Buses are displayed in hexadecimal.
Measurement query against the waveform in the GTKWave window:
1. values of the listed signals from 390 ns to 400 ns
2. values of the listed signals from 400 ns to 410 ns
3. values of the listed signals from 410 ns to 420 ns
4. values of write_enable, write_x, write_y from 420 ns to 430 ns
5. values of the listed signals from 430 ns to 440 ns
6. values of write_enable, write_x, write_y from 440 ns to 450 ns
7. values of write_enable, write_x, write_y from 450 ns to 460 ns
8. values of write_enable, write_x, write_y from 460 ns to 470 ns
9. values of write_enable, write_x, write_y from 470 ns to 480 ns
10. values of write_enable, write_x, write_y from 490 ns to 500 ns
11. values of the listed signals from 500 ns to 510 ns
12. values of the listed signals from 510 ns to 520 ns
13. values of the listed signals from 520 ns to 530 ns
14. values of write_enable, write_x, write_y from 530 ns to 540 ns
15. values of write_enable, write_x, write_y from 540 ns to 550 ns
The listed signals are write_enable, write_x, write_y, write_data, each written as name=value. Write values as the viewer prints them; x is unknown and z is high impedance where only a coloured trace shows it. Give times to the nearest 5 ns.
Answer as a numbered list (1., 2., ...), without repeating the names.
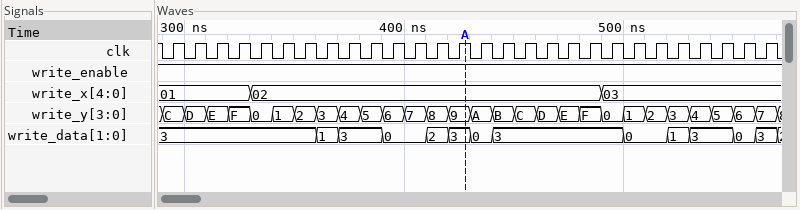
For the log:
1. write_enable=1, write_x=02, write_y=6, write_data=0
2. write_enable=1, write_x=02, write_y=7, write_data=0
3. write_enable=1, write_x=02, write_y=8, write_data=2
4. write_enable=1, write_x=02, write_y=9
5. write_enable=1, write_x=02, write_y=A, write_data=0
6. write_enable=1, write_x=02, write_y=B
7. write_enable=1, write_x=02, write_y=C
8. write_enable=1, write_x=02, write_y=D
9. write_enable=1, write_x=02, write_y=E
10. write_enable=1, write_x=03, write_y=0
11. write_enable=1, write_x=03, write_y=1, write_data=0
12. write_enable=1, write_x=03, write_y=2, write_data=0
13. write_enable=1, write_x=03, write_y=3, write_data=1
14. write_enable=1, write_x=03, write_y=4
15. write_enable=1, write_x=03, write_y=5
